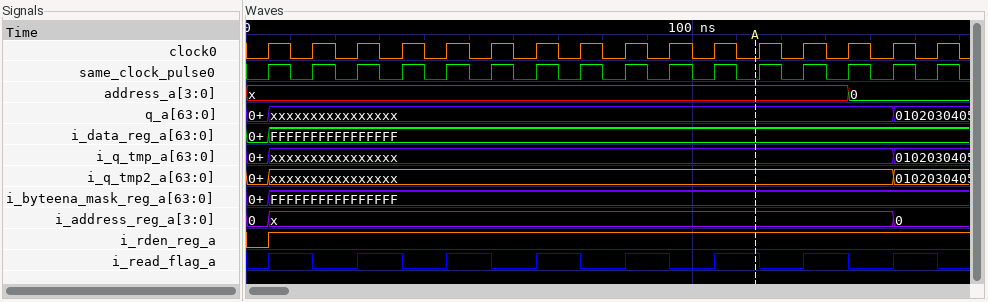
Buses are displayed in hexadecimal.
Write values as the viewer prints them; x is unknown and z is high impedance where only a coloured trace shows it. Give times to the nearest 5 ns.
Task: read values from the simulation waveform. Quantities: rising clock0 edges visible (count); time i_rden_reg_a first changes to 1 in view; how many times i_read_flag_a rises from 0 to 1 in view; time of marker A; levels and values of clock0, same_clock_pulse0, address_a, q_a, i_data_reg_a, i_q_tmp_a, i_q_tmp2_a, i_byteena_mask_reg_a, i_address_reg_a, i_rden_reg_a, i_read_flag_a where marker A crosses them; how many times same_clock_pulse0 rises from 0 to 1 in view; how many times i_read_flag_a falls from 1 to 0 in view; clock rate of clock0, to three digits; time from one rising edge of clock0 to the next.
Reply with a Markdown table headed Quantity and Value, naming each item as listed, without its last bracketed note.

| Quantity | Value |
|---|---|
| rising clock0 edges visible | 16 |
| time i_rden_reg_a first changes to 1 in view | 5 ns |
| how many times i_read_flag_a rises from 0 to 1 in view | 8 |
| time of marker A | 115 ns |
| levels and values of clock0, same_clock_pulse0, address_a, q_a, i_data_reg_a, i_q_tmp_a, i_q_tmp2_a, i_byteena_mask_reg_a, i_address_reg_a, i_rden_reg_a, i_read_flag_a where marker A crosses them | clock0=0, same_clock_pulse0=0, address_a=x, q_a=xxxxxxxxxxxxxxxx, i_data_reg_a=FFFFFFFFFFFFFFFF, i_q_tmp_a=xxxxxxxxxxxxxxxx, i_q_tmp2_a=xxxxxxxxxxxxxxxx, i_byteena_mask_reg_a=FFFFFFFFFFFFFFFF, i_address_reg_a=x, i_rden_reg_a=1, i_read_flag_a=1 |
| how many times same_clock_pulse0 rises from 0 to 1 in view | 16 |
| how many times i_read_flag_a falls from 1 to 0 in view | 8 |
| clock rate of clock0, to three digits | 100 MHz |
| time from one rising edge of clock0 to the next | 10 ns |
